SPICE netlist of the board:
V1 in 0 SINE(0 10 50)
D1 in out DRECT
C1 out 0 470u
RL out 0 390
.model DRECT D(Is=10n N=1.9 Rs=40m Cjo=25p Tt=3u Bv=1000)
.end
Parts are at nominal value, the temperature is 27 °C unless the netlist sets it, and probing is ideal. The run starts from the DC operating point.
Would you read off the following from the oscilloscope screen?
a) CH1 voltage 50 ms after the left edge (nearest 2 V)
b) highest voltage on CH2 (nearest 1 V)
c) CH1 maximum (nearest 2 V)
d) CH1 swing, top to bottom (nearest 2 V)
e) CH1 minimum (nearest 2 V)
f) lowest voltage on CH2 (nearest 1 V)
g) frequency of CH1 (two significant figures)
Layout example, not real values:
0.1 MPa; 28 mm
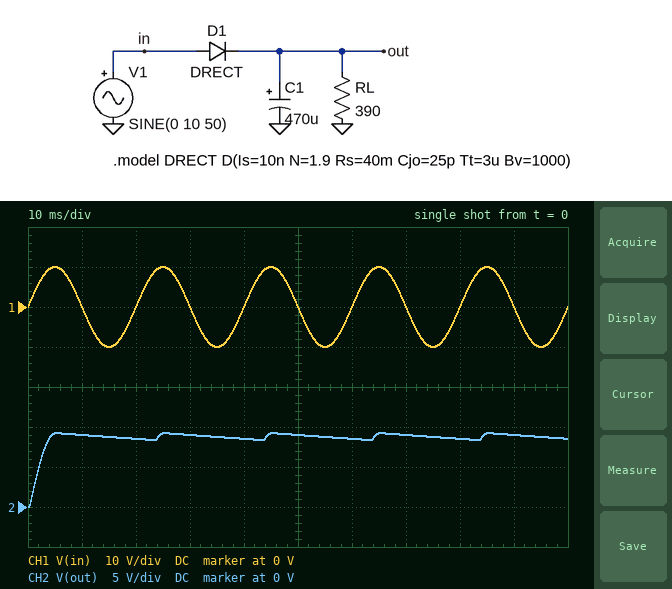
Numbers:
0 V; 9 V; 10 V; 20 V; -10 V; 0 V; 50 Hz
